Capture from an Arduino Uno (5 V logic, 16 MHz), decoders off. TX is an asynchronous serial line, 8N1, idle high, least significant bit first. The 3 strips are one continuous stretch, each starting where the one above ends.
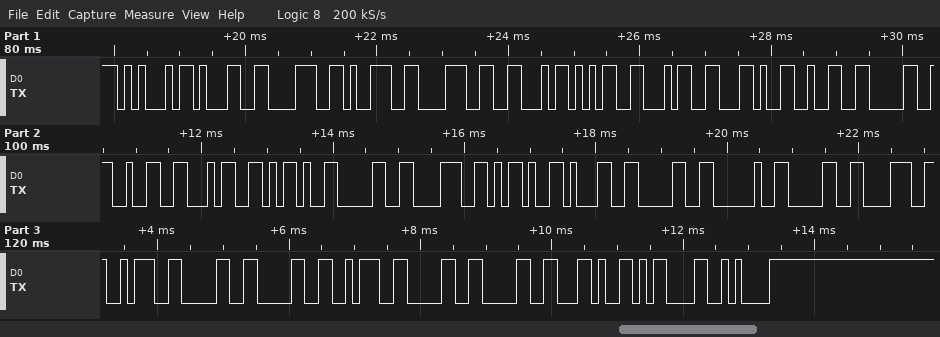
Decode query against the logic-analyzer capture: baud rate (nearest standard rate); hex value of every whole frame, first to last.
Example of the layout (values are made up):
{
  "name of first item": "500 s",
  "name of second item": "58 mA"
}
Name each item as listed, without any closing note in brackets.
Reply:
{
  "baud rate": "9600 baud",
  "hex value of every whole frame, first to last": "0x45 0x31 0x38 0x39 0x38 0x46 0x35 0x34 0x2C 0x32 0x30 0x32 0x34 0x2D 0x30 0x38 0x2D 0x31 0x30 0x20 0x30 0x38 0x3A 0x30 0x30 0x3A 0x30 0x30 0x2C 0x0D 0x0A"
}
